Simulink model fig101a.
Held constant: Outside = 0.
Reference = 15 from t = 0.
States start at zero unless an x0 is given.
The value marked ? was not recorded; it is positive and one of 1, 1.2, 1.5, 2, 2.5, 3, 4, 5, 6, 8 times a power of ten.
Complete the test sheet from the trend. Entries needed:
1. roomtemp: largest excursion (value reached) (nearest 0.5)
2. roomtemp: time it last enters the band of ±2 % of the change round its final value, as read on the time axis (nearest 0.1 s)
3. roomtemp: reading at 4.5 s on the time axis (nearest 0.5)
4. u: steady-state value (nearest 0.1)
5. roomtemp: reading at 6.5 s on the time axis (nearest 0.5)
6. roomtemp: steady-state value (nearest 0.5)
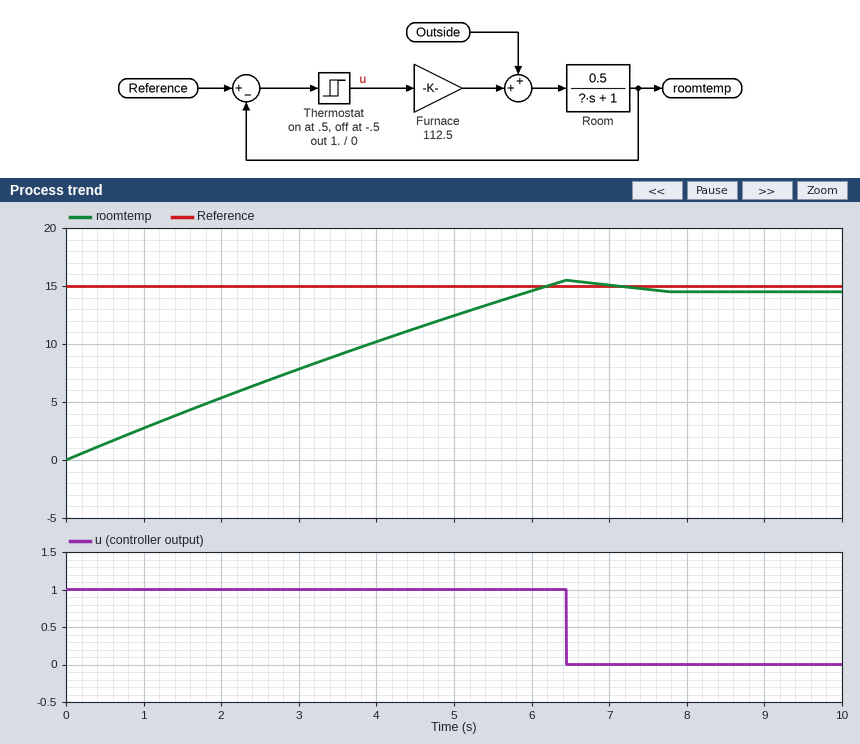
15.5
7.4 s
11.5
0.0
15.5
14.5
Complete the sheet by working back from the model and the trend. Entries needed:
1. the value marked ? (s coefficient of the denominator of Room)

20
